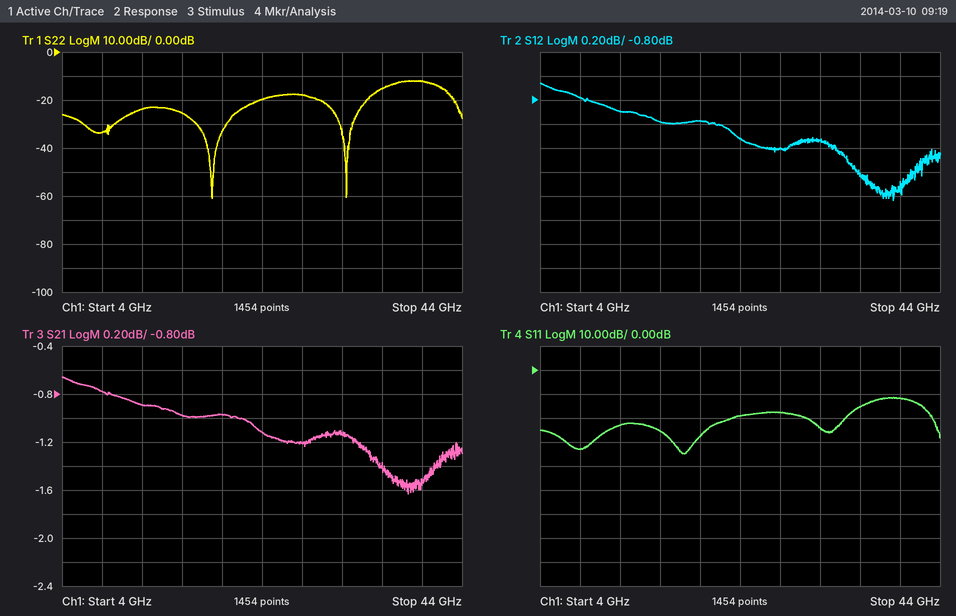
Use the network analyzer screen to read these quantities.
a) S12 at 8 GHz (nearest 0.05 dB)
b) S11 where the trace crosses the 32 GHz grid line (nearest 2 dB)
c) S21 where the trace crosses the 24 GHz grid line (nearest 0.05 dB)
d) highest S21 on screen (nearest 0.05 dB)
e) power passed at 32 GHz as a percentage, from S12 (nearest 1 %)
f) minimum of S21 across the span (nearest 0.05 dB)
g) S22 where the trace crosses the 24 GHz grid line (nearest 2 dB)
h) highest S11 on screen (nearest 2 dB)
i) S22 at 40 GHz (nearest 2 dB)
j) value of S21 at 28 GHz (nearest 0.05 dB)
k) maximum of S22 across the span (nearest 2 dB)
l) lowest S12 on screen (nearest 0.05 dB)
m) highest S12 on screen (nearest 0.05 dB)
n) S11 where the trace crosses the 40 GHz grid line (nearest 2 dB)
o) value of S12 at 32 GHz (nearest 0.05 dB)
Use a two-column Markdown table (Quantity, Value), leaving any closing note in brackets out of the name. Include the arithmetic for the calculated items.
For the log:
| Quantity | Value |
|---|---|
| S12 at 8 GHz | -0.80 dB |
| S11 where the trace crosses the 32 GHz grid line | -24 dB |
| S21 where the trace crosses the 24 GHz grid line | -1.10 dB |
| highest S21 on screen | -0.65 dB |
| power passed at 32 GHz as a percentage, from S12 | 10^(-1.15/10) ≈ 77 % |
| minimum of S21 across the span | -1.65 dB |
| S22 where the trace crosses the 24 GHz grid line | -20 dB |
| highest S11 on screen | -12 dB |
| S22 at 40 GHz | -12 dB |
| value of S21 at 28 GHz | -1.20 dB |
| maximum of S22 across the span | -12 dB |
| lowest S12 on screen | -1.65 dB |
| highest S12 on screen | -0.65 dB |
| S11 where the trace crosses the 40 GHz grid line | -12 dB |
| value of S12 at 32 GHz | -1.15 dB |
